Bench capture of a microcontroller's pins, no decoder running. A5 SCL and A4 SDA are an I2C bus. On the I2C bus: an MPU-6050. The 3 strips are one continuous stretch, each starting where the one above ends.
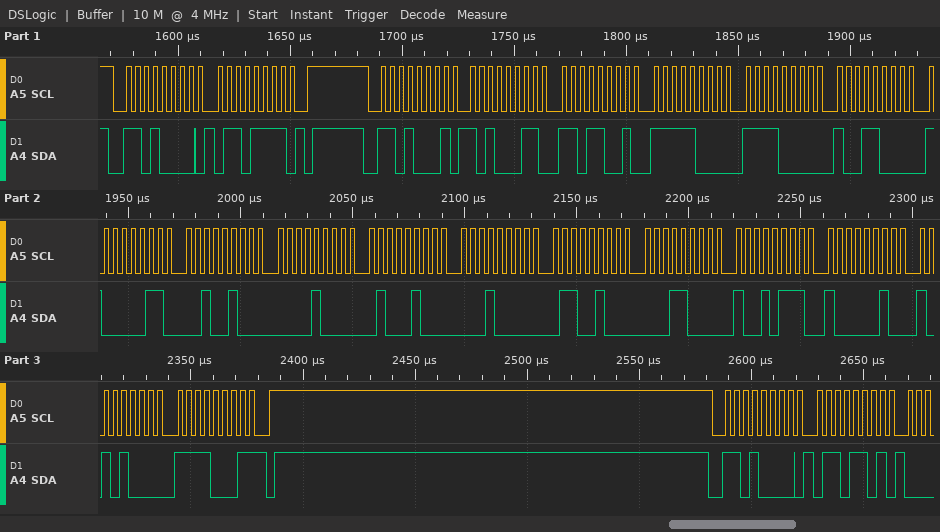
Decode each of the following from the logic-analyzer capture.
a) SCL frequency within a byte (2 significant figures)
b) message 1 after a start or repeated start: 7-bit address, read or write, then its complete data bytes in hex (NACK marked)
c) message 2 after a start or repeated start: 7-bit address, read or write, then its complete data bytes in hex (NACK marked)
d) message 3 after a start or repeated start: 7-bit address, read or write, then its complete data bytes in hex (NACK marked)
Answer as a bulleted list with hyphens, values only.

- 250 kHz
- 0x68 write: 6F
- 0x68 read: A3 D9 F8 F0 98 83 24 08 44 10 64 18 97 82 A8 F1 NACK
- 0x68 write: 6D
